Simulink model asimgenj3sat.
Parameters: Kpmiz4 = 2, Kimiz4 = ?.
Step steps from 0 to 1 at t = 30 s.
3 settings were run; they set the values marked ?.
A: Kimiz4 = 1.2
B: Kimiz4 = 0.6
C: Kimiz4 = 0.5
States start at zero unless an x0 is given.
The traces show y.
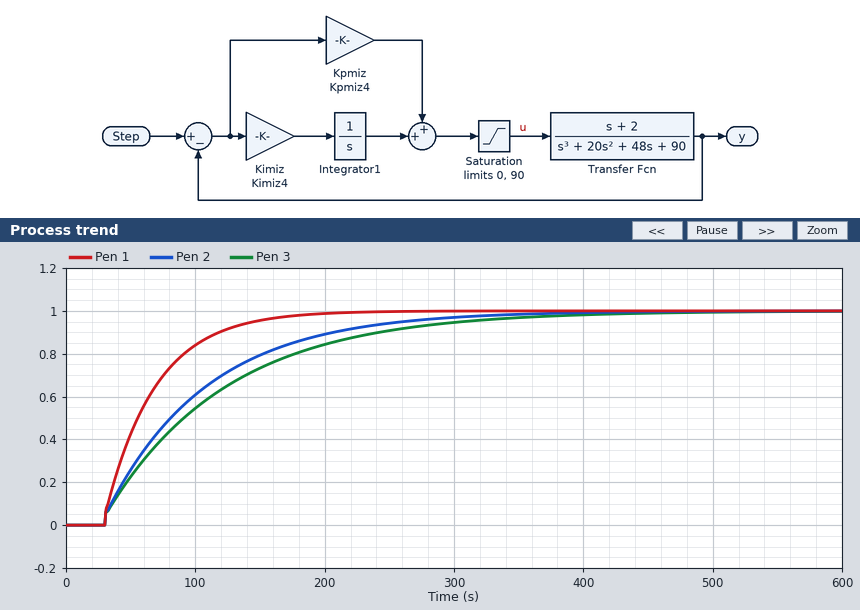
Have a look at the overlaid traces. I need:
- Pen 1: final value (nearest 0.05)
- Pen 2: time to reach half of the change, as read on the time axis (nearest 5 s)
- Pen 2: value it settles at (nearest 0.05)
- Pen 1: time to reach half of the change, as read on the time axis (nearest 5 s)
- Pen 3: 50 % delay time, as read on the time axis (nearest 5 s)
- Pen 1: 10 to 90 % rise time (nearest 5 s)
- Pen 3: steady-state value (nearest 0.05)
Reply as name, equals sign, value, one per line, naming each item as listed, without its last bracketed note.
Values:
Pen 1: final value = 1.00
Pen 2: time to reach half of the change, as read on the time axis = 80 s
Pen 2: value it settles at = 1.00
Pen 1: time to reach half of the change, as read on the time axis = 55 s
Pen 3: 50 % delay time, as read on the time axis = 90 s
Pen 1: 10 to 90 % rise time = 85 s
Pen 3: steady-state value = 1.00
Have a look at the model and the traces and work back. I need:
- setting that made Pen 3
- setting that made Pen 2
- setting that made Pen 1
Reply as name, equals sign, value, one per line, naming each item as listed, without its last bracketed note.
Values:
setting that made Pen 3 = C
setting that made Pen 2 = B
setting that made Pen 1 = A
